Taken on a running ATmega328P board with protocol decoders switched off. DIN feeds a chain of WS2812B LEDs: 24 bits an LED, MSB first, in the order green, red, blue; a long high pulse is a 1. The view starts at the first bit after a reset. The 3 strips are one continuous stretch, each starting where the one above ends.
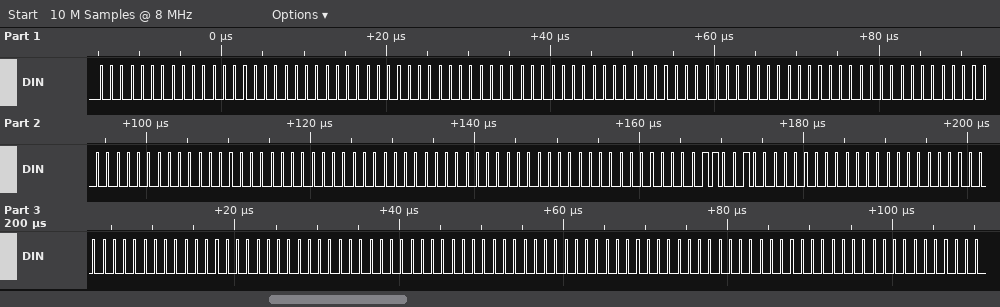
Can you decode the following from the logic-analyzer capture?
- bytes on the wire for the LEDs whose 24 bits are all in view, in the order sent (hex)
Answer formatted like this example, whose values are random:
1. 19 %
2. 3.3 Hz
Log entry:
1. 00 00 00 00 00 00 00 00 00 00 00 00 00 00 00 00 00 00 32 00 00 00 00 00 00 00 00 00 00 00
